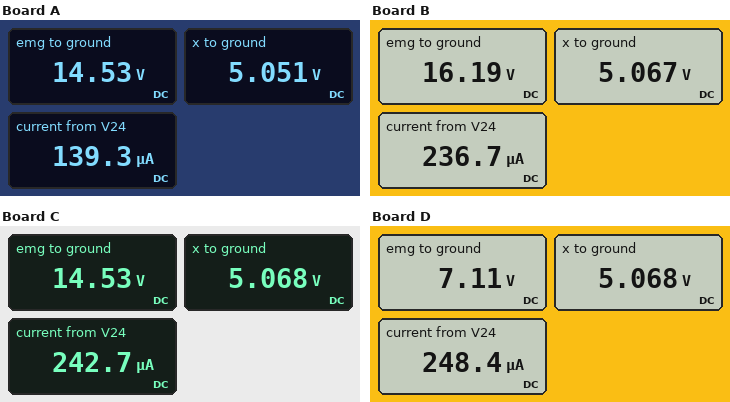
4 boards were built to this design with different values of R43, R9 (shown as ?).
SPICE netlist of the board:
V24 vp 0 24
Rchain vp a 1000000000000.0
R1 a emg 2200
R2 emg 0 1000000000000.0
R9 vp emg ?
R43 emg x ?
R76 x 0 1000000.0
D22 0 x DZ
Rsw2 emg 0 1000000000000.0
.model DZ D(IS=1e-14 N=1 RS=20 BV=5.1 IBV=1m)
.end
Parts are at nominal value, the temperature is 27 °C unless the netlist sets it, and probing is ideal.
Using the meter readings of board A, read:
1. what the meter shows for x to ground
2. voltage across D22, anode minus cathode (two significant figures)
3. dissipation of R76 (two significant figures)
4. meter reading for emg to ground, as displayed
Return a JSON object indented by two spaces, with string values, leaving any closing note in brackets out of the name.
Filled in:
{
  "what the meter shows for x to ground": "5.051 V",
  "voltage across D22, anode minus cathode": "-5.1 V",
  "dissipation of R76": "26 µW",
  "meter reading for emg to ground, as displayed": "14.53 V"
}
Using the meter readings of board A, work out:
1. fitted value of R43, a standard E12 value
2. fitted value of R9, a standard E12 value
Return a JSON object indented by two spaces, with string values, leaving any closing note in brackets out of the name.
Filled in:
{
  "fitted value of R43, a standard E12 value": "68 kΩ",
  "fitted value of R9, a standard E12 value": "68 kΩ"
}
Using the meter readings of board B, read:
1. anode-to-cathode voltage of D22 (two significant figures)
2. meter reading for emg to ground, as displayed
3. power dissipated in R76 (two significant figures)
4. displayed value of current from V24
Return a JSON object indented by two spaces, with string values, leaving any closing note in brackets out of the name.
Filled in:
{
  "anode-to-cathode voltage of D22": "-5.1 V",
  "meter reading for emg to ground, as displayed": "16.19 V",
  "power dissipated in R76": "26 µW",
  "displayed value of current from V24": "236.7 µA"
}
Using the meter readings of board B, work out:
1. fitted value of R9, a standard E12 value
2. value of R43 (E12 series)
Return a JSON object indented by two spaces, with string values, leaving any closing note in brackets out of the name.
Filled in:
{
  "fitted value of R9, a standard E12 value": "33 kΩ",
  "value of R43": "47 kΩ"
}
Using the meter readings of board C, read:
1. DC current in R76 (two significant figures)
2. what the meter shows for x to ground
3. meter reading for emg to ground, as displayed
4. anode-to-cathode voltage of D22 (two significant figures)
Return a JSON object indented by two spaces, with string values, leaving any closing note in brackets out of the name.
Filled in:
{
  "DC current in R76": "5.1 µA",
  "what the meter shows for x to ground": "5.068 V",
  "meter reading for emg to ground, as displayed": "14.53 V",
  "anode-to-cathode voltage of D22": "-5.1 V"
}
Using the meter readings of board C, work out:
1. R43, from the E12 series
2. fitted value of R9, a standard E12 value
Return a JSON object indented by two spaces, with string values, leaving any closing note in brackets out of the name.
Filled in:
{
  "R43, from the E12 series": "39 kΩ",
  "fitted value of R9, a standard E12 value": "39 kΩ"
}
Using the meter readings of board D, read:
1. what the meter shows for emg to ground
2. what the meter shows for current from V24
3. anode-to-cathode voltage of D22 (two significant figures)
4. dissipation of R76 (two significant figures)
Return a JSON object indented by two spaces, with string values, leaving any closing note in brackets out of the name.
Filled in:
{
  "what the meter shows for emg to ground": "7.11 V",
  "what the meter shows for current from V24": "248.4 µA",
  "anode-to-cathode voltage of D22": "-5.1 V",
  "dissipation of R76": "26 µW"
}
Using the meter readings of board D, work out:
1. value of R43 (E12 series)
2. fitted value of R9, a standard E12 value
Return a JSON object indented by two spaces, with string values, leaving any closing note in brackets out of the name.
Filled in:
{
  "value of R43": "8.2 kΩ",
  "fitted value of R9, a standard E12 value": "68 kΩ"
}
